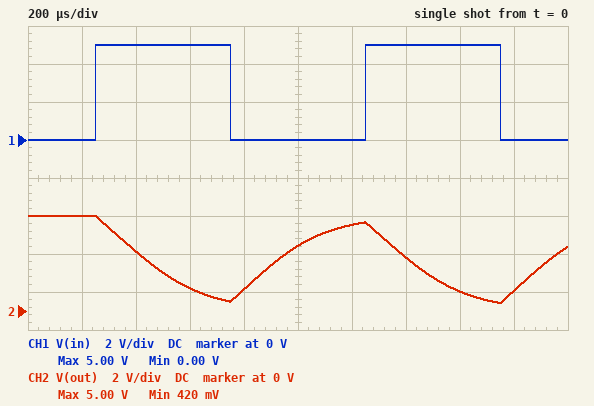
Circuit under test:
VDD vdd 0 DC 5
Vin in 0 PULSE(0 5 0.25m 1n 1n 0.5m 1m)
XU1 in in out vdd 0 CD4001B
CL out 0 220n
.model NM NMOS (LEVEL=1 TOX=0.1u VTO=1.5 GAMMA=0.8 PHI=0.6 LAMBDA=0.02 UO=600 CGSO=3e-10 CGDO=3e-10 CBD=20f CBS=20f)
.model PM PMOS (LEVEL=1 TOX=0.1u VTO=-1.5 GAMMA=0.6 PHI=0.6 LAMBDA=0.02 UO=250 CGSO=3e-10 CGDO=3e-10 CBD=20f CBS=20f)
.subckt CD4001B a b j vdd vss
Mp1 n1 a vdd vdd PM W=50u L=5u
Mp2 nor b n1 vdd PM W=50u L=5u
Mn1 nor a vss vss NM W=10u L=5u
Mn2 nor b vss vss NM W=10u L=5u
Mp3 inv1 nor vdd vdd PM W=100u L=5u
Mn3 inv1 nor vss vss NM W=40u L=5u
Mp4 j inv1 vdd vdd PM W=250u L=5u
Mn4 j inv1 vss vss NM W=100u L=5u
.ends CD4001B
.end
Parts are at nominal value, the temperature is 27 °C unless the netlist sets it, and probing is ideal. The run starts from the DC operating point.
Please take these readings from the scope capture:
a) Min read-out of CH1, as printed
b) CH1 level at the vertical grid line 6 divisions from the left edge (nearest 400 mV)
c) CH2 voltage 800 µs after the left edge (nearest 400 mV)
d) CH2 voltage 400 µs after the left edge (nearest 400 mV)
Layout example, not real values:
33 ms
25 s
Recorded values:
0.00 V
0 V
1.2 V
3.2 V
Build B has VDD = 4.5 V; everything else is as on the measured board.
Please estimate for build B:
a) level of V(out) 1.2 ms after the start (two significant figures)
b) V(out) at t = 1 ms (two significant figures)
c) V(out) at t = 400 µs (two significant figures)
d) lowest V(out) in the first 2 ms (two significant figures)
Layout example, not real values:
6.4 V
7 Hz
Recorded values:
3.9 V
2.9 V
3.1 V
580 mV
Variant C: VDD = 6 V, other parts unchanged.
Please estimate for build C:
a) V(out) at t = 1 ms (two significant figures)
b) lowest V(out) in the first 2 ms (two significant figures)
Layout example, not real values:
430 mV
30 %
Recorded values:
4.7 V
190 mV
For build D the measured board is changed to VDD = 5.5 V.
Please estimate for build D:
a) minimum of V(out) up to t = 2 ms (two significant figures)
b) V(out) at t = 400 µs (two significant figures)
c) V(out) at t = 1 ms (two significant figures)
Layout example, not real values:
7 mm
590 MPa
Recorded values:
290 mV
3.1 V
4.0 V
